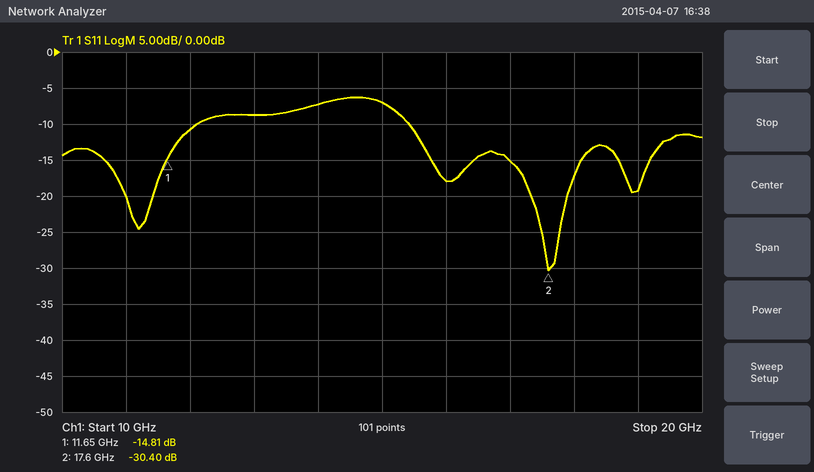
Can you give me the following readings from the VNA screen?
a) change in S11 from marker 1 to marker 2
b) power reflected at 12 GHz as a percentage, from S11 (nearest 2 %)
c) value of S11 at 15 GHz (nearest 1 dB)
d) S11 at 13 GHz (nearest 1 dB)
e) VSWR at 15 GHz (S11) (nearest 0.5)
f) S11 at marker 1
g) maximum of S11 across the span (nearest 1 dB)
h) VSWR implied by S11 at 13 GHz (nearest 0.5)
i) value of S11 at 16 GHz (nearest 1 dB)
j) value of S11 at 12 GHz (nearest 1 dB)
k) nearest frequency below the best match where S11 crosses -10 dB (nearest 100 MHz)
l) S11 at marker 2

-15.59 dB
8 %
-7 dB
-9 dB
2.5
-14.81 dB
-6 dB
2.0
-18 dB
-11 dB
15.4 GHz
-30.40 dB
